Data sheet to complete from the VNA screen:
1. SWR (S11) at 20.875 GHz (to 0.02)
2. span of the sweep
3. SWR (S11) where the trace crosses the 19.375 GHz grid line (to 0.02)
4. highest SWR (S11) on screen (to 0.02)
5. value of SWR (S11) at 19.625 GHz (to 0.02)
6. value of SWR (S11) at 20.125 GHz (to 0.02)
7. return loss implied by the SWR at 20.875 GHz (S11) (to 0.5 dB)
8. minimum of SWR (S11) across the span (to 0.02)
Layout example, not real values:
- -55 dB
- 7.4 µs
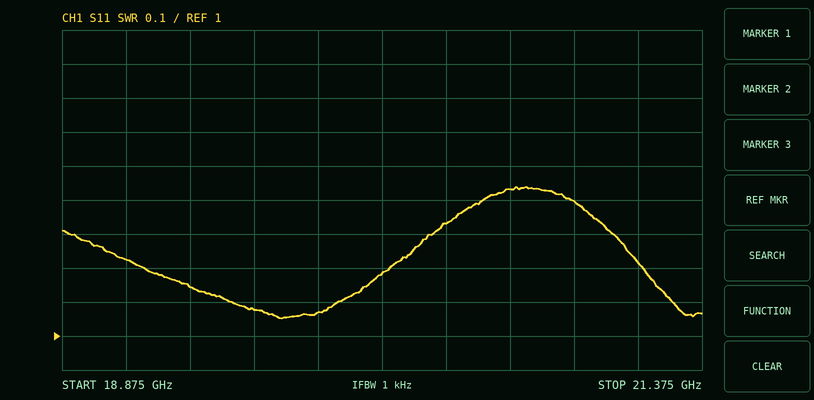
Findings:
- 1.40
- 2.5 GHz
- 1.14
- 1.44
- 1.08
- 1.18
- 15.5 dB
- 1.06
